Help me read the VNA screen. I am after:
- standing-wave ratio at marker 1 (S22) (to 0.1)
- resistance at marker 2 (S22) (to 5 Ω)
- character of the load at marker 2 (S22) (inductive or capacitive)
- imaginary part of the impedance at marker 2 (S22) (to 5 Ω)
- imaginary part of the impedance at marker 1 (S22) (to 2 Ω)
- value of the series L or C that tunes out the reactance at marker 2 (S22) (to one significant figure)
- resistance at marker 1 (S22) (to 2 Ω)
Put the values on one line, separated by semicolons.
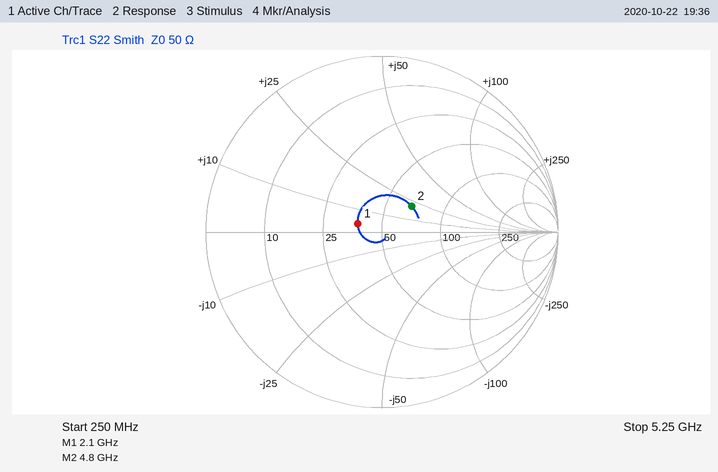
1.3; 65 Ω; inductive; +20 Ω; +4 Ω; 2 pF; 38 Ω
